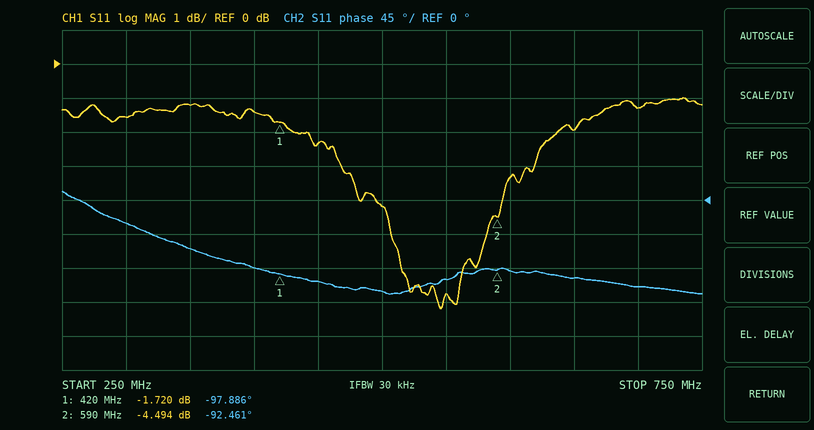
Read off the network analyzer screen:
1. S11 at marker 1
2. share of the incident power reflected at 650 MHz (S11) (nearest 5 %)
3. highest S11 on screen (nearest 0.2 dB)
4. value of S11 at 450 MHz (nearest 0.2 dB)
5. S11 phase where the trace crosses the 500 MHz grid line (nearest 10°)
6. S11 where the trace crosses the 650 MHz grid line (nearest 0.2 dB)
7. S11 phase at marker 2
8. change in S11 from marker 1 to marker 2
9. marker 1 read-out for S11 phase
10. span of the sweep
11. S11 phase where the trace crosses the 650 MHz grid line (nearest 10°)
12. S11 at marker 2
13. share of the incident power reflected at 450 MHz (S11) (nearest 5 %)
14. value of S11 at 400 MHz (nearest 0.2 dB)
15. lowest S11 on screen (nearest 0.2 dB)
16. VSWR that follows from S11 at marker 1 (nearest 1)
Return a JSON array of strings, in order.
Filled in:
["-1.720 dB", "65 %", "-1.0 dB", "-2.4 dB", "-120°", "-2.0 dB", "-92.461°", "-2.774 dB", "-97.886°", "500 MHz", "-100°", "-4.494 dB", "60 %", "-1.4 dB", "-7.2 dB", "10"]
